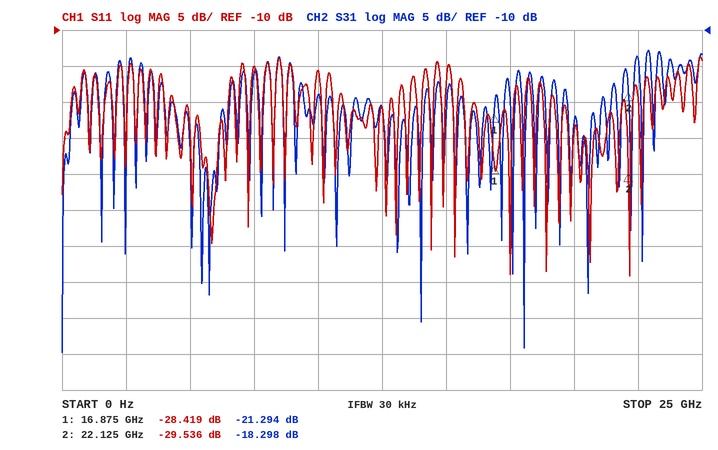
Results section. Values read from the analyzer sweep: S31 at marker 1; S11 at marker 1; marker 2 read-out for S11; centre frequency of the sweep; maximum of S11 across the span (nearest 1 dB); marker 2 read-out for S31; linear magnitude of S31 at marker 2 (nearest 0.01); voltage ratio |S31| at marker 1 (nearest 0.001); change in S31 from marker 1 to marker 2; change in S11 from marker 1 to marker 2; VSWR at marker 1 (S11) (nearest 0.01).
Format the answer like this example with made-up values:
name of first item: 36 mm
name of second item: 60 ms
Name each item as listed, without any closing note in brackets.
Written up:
S31 at marker 1: -21.294 dB
S11 at marker 1: -28.419 dB
marker 2 read-out for S11: -29.536 dB
centre frequency of the sweep: 12.5 GHz
maximum of S11 across the span: -14 dB
marker 2 read-out for S31: -18.298 dB
linear magnitude of S31 at marker 2: 0.12
voltage ratio |S31| at marker 1: 0.086
change in S31 from marker 1 to marker 2: 2.996 dB
change in S11 from marker 1 to marker 2: -1.117 dB
VSWR at marker 1 (S11): 1.08
